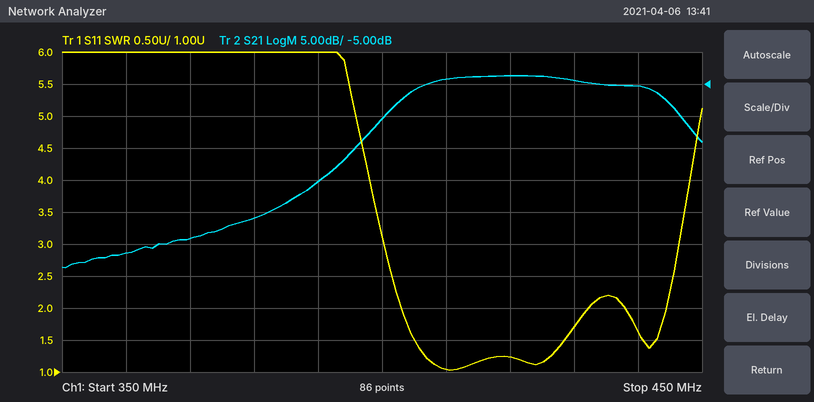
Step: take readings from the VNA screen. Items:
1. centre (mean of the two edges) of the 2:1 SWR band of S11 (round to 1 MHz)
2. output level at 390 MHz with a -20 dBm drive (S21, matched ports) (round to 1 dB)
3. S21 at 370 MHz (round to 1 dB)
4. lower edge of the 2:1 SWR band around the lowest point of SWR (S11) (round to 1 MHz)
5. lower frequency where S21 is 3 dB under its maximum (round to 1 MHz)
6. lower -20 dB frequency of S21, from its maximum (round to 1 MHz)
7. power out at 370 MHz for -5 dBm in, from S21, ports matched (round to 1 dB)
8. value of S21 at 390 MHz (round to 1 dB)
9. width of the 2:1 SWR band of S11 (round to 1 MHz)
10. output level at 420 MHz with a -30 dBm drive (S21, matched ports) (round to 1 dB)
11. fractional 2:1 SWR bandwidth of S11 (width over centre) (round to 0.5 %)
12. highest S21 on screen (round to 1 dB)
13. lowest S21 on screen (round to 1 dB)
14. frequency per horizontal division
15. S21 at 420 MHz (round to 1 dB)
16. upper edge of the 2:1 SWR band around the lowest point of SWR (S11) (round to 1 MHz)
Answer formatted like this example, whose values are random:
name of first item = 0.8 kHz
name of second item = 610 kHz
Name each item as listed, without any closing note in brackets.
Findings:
centre (mean of the two edges) of the 2:1 SWR band of S11 = 418 MHz
output level at 390 MHz with a -20 dBm drive (S21, matched ports) = -40 dBm
S21 at 370 MHz = -29 dB
lower edge of the 2:1 SWR band around the lowest point of SWR (S11) = 403 MHz
lower frequency where S21 is 3 dB under its maximum = 404 MHz
lower -20 dB frequency of S21, from its maximum = 385 MHz
power out at 370 MHz for -5 dBm in, from S21, ports matched = -34 dBm
value of S21 at 390 MHz = -20 dB
width of the 2:1 SWR band of S11 = 29 MHz
output level at 420 MHz with a -30 dBm drive (S21, matched ports) = -34 dBm
fractional 2:1 SWR bandwidth of S11 (width over centre) = 7.0 %
highest S21 on screen = -4 dB
lowest S21 on screen = -34 dB
frequency per horizontal division = 10 MHz
S21 at 420 MHz = -4 dB
upper edge of the 2:1 SWR band around the lowest point of SWR (S11) = 432 MHz
